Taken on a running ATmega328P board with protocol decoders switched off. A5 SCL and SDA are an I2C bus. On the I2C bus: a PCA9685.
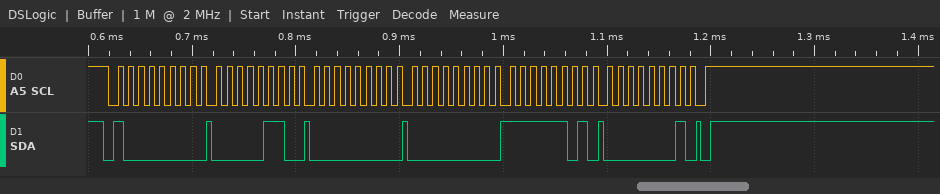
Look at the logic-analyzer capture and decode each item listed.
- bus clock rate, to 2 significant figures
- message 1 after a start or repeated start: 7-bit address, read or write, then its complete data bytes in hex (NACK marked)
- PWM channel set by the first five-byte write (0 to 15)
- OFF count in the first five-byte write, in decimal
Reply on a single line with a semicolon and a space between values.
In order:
100 kHz; 0x40 write: 06 00 00 FD 01; 0; 509
